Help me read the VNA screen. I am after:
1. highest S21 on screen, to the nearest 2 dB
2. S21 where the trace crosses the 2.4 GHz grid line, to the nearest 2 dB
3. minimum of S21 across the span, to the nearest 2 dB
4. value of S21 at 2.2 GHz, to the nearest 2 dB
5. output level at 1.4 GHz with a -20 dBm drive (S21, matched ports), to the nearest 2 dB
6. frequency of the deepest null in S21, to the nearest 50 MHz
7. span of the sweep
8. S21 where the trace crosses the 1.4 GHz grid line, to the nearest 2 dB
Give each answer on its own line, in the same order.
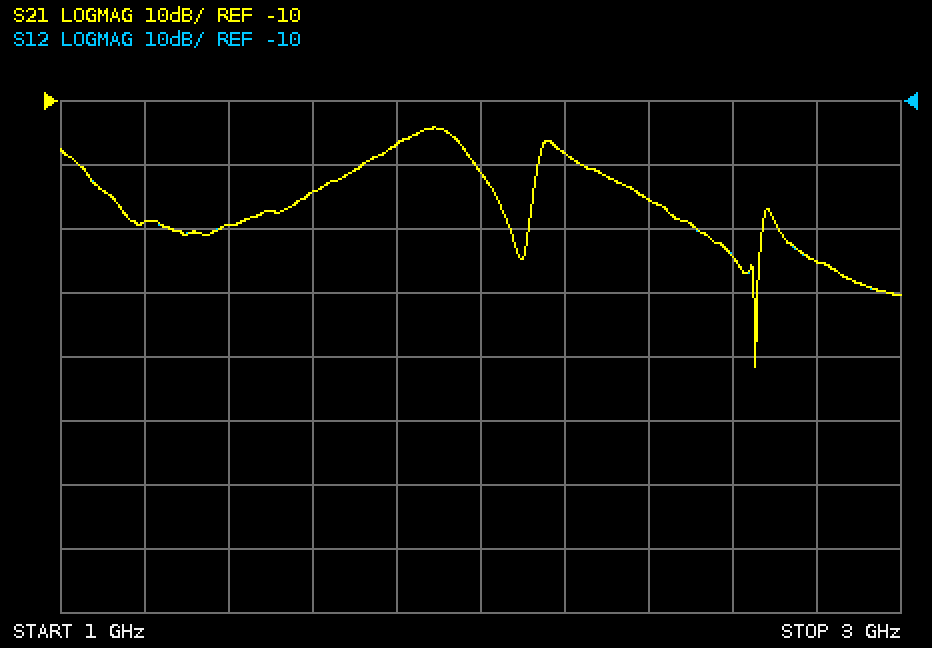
-14 dB
-26 dB
-52 dB
-18 dB
-50 dBm
2.65 GHz
2 GHz
-30 dB
